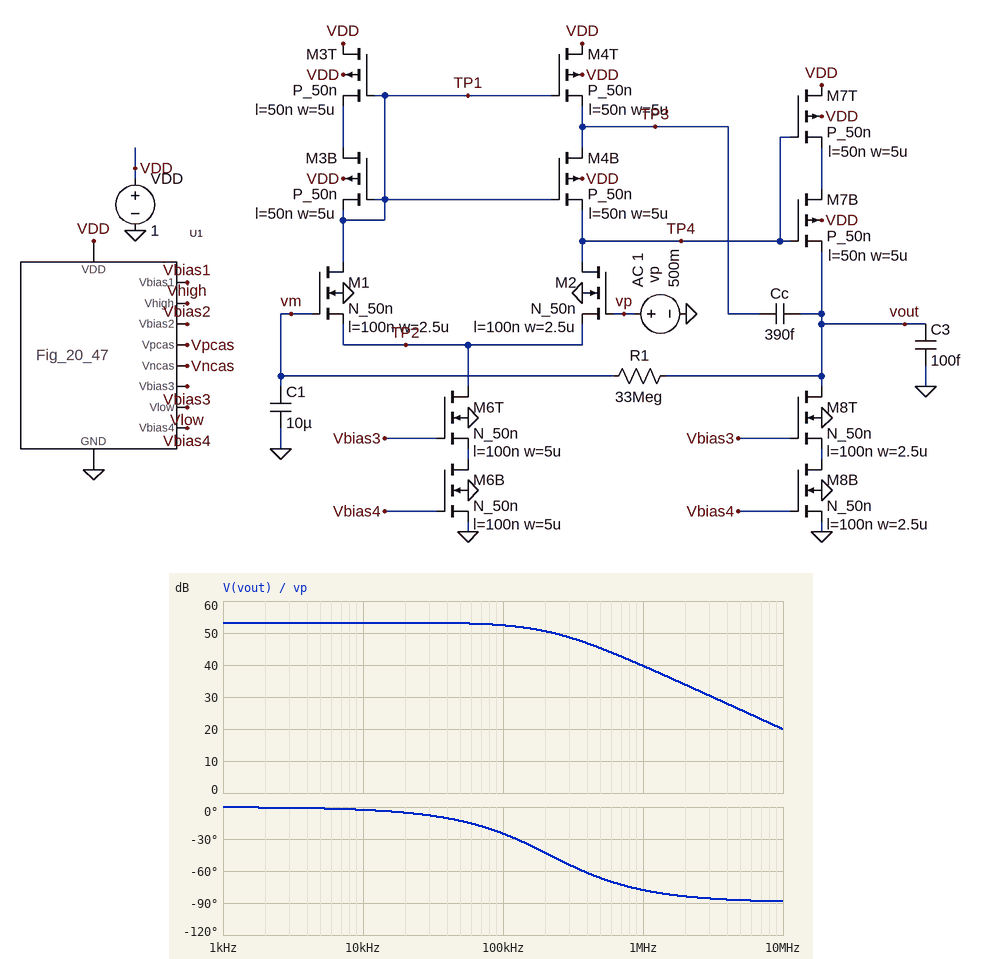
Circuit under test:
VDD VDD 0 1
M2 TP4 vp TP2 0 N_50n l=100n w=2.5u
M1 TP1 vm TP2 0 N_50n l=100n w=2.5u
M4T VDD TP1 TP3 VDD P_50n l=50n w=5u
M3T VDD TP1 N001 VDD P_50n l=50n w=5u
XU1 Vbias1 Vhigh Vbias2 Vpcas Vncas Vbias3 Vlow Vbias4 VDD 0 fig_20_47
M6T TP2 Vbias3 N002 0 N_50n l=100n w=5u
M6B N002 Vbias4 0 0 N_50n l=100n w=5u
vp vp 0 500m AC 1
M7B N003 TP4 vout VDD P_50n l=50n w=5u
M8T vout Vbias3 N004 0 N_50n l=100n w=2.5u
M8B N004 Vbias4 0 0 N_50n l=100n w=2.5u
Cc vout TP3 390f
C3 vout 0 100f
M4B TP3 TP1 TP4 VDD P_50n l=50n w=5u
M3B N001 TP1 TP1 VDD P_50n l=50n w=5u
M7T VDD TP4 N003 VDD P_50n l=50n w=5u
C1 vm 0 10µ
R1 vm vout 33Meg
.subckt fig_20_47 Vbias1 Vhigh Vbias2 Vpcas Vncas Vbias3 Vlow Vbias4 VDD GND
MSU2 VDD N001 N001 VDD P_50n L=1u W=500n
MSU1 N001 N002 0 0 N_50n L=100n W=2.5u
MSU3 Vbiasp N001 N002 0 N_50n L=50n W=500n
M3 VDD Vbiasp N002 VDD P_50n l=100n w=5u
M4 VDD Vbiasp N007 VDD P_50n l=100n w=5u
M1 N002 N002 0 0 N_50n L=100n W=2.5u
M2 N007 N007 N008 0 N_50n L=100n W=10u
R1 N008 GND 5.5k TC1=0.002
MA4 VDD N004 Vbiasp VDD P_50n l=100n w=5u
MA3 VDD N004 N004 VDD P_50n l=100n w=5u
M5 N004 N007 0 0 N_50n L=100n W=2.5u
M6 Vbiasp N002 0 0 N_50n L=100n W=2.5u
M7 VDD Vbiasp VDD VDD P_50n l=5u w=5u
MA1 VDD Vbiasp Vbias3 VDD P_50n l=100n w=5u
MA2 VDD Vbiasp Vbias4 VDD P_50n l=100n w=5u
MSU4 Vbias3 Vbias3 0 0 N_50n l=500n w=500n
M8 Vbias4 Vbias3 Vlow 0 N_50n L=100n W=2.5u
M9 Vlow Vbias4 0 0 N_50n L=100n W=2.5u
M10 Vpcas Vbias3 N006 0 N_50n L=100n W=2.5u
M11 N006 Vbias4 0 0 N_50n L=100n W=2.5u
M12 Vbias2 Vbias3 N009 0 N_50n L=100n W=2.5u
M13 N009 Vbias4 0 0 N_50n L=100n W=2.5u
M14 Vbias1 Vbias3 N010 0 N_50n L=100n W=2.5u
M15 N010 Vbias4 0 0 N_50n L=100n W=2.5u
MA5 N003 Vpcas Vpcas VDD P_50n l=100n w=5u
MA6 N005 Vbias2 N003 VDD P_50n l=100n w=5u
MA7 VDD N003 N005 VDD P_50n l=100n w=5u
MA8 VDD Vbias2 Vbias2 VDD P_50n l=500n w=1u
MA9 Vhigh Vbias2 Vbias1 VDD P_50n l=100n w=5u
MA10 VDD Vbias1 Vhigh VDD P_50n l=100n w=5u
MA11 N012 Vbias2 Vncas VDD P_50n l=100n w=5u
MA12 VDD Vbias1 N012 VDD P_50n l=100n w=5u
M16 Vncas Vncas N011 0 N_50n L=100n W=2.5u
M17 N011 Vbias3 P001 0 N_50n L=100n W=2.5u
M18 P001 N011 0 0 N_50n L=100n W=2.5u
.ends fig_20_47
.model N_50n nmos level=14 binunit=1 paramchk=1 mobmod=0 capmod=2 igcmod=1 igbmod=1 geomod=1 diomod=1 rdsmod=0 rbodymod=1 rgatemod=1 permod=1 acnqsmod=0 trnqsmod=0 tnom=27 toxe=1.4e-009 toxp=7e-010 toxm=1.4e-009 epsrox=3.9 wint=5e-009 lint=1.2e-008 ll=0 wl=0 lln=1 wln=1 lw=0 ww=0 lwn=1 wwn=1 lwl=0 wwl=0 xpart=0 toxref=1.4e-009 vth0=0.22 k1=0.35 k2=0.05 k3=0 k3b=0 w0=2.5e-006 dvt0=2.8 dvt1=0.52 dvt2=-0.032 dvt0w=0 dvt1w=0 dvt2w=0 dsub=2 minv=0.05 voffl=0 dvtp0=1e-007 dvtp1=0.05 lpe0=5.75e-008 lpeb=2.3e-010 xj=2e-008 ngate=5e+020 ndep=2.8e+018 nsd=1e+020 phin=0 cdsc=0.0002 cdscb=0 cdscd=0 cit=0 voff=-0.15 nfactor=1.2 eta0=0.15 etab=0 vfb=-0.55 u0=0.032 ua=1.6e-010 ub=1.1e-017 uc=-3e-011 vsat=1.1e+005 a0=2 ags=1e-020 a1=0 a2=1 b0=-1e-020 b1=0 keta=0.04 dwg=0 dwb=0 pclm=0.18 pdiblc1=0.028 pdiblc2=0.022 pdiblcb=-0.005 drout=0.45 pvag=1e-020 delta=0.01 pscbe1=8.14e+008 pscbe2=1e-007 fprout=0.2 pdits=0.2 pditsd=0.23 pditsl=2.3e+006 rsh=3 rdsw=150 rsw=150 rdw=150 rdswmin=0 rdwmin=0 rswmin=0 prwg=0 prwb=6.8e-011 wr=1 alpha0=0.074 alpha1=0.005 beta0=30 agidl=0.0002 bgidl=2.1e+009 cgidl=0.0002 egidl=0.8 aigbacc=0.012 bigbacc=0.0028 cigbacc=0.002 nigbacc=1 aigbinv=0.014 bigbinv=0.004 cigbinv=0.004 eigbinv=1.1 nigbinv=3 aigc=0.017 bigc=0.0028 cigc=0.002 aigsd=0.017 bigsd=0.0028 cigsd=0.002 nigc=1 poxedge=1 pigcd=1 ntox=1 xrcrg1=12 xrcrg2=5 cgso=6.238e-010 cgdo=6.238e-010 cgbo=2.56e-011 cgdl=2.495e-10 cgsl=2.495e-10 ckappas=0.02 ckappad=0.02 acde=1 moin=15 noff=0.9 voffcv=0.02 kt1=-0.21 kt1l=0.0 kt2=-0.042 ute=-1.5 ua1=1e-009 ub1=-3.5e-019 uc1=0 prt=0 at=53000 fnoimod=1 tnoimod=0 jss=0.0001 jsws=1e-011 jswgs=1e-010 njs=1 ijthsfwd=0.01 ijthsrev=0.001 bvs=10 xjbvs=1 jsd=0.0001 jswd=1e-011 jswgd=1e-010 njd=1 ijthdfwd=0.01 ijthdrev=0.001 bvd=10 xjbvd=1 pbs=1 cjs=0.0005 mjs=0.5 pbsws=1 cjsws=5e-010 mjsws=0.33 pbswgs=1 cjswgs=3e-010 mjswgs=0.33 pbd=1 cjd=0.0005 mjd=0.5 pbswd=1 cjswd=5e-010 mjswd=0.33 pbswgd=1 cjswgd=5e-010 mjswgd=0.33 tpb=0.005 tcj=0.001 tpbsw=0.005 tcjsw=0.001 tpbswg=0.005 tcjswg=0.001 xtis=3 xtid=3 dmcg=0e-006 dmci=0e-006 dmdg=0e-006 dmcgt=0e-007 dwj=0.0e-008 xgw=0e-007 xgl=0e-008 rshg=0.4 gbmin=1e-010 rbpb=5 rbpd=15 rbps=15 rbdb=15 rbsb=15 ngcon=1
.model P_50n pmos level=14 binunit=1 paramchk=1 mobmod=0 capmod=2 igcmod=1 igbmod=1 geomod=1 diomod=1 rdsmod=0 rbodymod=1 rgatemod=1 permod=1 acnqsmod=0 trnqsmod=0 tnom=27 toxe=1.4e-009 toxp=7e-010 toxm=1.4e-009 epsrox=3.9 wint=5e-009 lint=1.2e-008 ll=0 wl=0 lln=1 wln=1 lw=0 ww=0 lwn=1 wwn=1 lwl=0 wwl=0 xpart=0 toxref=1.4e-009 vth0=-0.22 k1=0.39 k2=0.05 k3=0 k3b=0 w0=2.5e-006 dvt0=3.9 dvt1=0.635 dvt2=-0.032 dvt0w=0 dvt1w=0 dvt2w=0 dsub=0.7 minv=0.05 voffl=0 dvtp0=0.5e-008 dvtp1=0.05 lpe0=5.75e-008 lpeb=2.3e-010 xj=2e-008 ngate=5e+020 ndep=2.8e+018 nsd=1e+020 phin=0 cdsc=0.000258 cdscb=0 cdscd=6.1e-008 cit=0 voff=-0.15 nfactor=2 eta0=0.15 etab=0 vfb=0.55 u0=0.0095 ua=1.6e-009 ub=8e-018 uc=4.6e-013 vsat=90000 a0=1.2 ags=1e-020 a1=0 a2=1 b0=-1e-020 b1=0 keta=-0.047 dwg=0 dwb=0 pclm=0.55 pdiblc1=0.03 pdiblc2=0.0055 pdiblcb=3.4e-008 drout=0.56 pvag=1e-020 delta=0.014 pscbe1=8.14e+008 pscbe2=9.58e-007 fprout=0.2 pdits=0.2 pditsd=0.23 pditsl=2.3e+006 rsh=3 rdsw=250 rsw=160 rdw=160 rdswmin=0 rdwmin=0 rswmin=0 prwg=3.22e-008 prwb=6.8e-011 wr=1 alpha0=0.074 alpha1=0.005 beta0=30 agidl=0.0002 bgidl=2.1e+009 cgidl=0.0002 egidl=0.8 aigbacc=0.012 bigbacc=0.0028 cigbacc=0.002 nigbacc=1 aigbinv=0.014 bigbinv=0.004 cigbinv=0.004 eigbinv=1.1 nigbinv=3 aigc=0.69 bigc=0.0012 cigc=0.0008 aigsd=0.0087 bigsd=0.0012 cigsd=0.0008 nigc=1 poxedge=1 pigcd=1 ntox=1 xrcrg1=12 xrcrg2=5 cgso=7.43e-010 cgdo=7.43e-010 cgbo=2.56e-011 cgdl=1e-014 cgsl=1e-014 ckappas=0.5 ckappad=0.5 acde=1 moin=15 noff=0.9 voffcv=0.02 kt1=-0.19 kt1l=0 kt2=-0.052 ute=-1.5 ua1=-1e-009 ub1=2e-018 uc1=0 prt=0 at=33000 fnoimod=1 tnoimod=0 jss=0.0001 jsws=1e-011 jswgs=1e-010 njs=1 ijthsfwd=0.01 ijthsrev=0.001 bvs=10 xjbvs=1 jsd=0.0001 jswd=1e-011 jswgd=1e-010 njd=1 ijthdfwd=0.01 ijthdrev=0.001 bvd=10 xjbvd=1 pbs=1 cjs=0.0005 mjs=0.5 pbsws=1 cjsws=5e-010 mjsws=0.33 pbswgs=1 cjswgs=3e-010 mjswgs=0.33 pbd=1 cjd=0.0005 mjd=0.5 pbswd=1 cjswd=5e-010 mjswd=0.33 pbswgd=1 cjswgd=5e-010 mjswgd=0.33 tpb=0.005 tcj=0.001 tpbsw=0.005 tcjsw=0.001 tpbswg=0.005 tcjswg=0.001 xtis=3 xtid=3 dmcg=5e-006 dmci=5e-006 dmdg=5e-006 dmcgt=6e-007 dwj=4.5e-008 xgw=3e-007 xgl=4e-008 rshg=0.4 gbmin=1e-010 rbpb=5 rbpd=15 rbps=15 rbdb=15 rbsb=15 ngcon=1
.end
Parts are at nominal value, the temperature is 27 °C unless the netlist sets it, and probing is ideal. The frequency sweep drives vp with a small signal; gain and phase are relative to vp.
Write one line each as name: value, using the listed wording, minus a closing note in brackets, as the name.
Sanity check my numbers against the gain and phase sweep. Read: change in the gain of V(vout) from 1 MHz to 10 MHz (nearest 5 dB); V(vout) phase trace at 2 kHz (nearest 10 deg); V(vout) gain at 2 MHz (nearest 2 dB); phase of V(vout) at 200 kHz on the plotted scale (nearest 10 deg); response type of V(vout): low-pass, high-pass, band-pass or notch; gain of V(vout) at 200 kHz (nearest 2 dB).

change in the gain of V(vout) from 1 MHz to 10 MHz: -20 dB
V(vout) phase trace at 2 kHz: 0 deg
V(vout) gain at 2 MHz: 34 dB
phase of V(vout) at 200 kHz on the plotted scale: -40 deg
response type of V(vout): low-pass, high-pass, band-pass or notch: low-pass
gain of V(vout) at 200 kHz: 50 dB
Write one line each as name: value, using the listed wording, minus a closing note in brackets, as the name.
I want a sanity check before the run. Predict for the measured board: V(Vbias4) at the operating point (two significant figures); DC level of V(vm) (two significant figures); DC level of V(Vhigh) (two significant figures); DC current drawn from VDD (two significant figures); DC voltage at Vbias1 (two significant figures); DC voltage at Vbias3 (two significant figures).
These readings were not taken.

V(Vbias4) at the operating point: 360 mV
DC level of V(vm): 500 mV
DC level of V(Vhigh): 790 mV
DC current drawn from VDD: 140 µA
DC voltage at Vbias1: 640 mV
DC voltage at Vbias3: 540 mV
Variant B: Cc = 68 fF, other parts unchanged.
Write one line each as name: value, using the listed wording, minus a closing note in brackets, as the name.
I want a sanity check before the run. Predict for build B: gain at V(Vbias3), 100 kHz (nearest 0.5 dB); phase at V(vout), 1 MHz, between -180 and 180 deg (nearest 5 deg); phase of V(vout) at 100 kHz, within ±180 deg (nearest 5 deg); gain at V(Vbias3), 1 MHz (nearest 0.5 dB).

gain at V(Vbias3), 100 kHz: -36.5 dB
phase at V(vout), 1 MHz, between -180 and 180 deg: -45 deg
phase of V(vout) at 100 kHz, within ±180 deg: -5 deg
gain at V(Vbias3), 1 MHz: -20.0 dB
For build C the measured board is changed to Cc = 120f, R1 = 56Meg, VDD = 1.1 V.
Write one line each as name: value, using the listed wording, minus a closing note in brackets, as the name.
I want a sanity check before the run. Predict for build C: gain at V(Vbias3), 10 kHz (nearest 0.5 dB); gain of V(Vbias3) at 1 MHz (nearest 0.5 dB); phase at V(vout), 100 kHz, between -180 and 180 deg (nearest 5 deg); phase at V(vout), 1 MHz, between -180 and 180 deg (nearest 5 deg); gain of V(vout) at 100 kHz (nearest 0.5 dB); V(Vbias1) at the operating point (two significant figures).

gain at V(Vbias3), 10 kHz: -55.0 dB
gain of V(Vbias3) at 1 MHz: -22.0 dB
phase at V(vout), 100 kHz, between -180 and 180 deg: -10 deg
phase at V(vout), 1 MHz, between -180 and 180 deg: -60 deg
gain of V(vout) at 100 kHz: 54.0 dB
V(Vbias1) at the operating point: 740 mV
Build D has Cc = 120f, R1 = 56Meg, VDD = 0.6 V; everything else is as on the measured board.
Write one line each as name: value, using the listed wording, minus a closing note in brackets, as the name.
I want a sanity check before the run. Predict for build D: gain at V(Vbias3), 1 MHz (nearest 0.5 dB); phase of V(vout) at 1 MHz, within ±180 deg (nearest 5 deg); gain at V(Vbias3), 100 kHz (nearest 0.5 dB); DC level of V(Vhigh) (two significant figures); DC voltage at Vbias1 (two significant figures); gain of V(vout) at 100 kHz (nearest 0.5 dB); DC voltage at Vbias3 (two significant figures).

gain at V(Vbias3), 1 MHz: -41.0 dB
phase of V(vout) at 1 MHz, within ±180 deg: -10 deg
gain at V(Vbias3), 100 kHz: -61.0 dB
DC level of V(Vhigh): 450 mV
DC voltage at Vbias1: 240 mV
gain of V(vout) at 100 kHz: 33.0 dB
DC voltage at Vbias3: 520 mV
